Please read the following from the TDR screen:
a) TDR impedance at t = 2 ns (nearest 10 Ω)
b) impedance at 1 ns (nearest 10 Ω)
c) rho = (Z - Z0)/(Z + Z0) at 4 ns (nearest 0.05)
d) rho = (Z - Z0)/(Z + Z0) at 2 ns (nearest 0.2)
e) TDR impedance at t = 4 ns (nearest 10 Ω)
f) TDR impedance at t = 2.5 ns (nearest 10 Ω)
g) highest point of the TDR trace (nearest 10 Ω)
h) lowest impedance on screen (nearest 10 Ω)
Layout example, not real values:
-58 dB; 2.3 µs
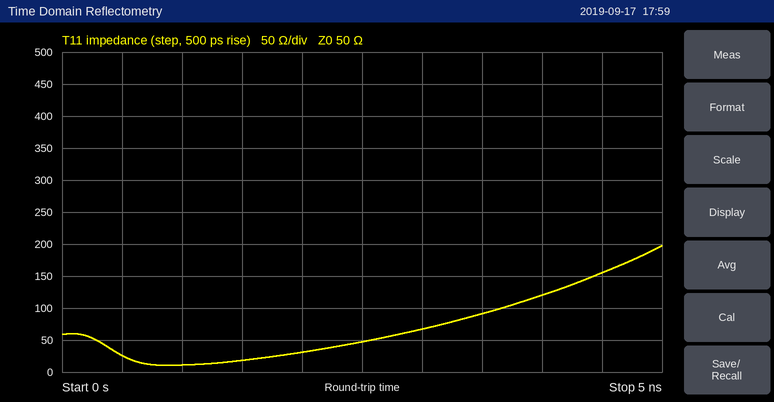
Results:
30 Ω; 10 Ω; +0.40; -0.2; 120 Ω; 50 Ω; 200 Ω; 10 Ω
